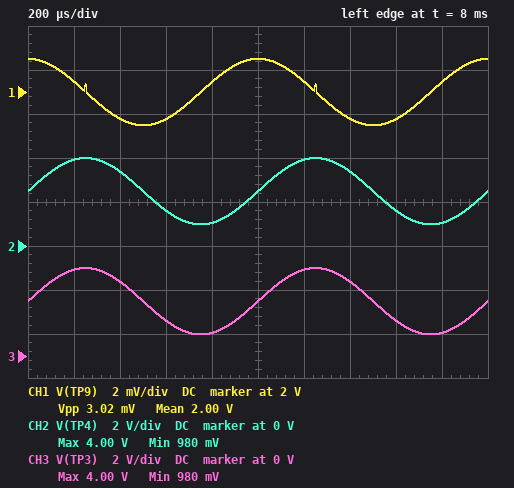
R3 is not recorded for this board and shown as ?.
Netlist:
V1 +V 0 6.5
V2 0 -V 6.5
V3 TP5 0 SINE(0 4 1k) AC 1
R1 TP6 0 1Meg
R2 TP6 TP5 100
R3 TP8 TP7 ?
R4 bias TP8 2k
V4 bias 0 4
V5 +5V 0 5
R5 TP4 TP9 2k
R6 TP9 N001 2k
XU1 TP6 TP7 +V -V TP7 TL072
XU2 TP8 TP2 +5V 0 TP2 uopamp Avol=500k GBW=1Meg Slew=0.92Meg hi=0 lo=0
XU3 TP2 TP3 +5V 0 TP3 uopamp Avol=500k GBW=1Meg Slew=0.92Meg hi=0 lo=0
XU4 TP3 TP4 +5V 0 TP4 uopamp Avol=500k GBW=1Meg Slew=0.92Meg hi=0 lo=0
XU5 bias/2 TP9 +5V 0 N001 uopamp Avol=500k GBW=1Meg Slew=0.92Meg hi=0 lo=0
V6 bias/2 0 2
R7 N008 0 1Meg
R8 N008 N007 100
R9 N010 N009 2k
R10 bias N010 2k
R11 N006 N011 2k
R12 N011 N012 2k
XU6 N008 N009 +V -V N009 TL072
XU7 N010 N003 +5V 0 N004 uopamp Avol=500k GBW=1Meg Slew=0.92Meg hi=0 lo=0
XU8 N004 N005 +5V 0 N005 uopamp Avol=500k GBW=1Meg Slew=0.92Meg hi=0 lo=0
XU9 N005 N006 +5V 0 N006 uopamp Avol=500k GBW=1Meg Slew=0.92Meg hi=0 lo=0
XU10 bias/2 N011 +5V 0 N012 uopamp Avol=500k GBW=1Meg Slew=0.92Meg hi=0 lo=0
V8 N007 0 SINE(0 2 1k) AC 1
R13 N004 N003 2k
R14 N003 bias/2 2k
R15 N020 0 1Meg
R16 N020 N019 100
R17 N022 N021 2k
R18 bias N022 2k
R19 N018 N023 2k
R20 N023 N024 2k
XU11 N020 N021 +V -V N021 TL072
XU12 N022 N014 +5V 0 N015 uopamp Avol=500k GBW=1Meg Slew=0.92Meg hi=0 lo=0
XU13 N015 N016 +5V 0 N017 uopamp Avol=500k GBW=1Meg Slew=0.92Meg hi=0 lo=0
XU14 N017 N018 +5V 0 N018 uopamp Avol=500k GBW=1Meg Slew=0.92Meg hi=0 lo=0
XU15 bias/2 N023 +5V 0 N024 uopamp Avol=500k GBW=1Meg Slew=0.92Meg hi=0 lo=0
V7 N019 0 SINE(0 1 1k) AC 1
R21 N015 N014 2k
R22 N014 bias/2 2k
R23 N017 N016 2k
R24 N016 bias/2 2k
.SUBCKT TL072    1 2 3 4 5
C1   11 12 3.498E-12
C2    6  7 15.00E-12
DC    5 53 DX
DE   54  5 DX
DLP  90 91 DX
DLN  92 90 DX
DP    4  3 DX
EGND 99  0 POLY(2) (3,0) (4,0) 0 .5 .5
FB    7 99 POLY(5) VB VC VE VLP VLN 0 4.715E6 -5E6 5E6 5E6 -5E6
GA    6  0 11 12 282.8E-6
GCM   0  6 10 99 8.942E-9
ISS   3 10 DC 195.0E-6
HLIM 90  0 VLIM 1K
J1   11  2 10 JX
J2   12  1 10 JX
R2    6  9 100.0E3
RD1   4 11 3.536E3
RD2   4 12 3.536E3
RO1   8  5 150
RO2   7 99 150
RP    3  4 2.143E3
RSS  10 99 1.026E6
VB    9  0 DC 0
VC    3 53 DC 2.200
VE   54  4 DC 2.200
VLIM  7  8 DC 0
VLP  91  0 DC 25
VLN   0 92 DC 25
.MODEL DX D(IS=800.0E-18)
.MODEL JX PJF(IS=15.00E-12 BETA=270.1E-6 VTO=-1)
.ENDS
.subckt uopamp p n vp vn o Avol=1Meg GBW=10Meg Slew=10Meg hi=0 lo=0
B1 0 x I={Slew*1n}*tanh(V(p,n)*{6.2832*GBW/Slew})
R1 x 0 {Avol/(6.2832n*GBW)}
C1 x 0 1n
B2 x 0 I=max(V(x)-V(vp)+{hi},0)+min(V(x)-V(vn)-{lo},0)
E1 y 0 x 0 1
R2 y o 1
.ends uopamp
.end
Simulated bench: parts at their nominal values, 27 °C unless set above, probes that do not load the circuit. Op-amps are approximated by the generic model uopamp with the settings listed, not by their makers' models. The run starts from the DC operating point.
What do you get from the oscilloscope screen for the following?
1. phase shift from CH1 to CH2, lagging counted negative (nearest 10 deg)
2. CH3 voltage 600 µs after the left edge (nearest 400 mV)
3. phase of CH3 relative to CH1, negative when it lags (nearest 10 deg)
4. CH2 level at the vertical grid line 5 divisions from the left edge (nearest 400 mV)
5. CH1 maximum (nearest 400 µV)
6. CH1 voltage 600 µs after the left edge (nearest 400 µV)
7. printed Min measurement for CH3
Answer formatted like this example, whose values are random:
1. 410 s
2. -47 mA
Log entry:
1. -90 deg
2. 1.6 V
3. -90 deg
4. 2.4 V
5. 2.0016 V
6. 1.9988 V
7. 980 mV
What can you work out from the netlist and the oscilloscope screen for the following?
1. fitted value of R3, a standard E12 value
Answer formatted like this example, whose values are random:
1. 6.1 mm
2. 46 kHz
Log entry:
1. 3.3 kΩ
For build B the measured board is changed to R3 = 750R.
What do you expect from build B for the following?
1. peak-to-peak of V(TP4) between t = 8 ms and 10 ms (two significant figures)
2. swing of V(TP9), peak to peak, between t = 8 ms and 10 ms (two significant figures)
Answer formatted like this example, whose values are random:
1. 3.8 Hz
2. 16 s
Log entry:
1. 4.0 V
2. 5.8 mV
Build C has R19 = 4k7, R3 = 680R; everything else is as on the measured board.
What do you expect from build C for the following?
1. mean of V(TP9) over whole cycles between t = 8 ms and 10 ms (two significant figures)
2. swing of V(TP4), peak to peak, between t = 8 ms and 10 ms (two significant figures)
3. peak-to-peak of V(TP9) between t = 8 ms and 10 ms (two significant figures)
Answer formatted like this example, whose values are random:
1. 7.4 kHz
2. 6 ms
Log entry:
1. 2.0 V
2. 4.0 V
3. 6.0 mV
